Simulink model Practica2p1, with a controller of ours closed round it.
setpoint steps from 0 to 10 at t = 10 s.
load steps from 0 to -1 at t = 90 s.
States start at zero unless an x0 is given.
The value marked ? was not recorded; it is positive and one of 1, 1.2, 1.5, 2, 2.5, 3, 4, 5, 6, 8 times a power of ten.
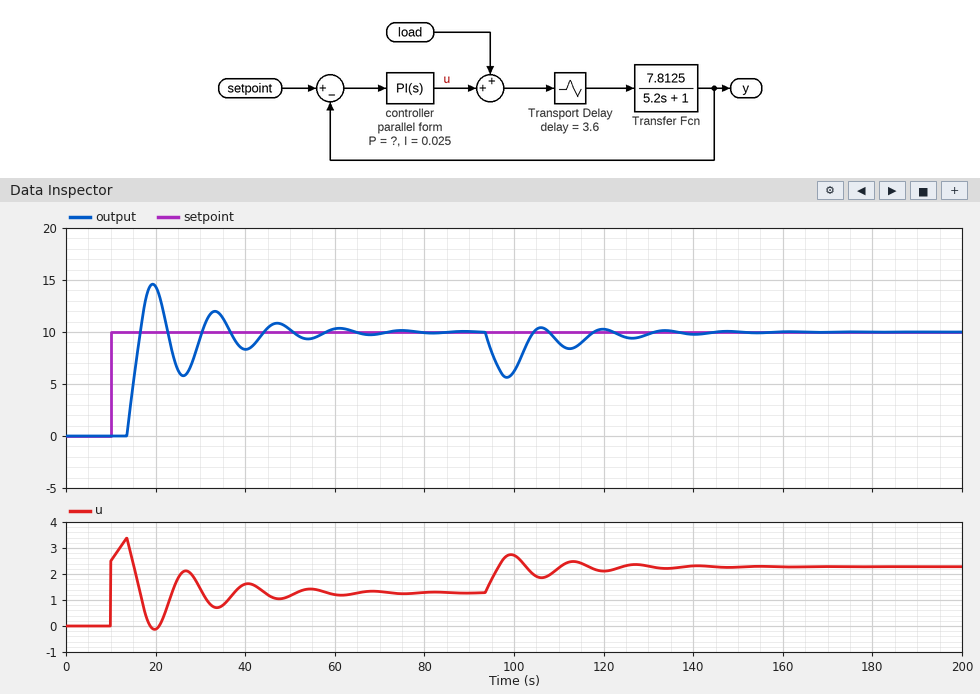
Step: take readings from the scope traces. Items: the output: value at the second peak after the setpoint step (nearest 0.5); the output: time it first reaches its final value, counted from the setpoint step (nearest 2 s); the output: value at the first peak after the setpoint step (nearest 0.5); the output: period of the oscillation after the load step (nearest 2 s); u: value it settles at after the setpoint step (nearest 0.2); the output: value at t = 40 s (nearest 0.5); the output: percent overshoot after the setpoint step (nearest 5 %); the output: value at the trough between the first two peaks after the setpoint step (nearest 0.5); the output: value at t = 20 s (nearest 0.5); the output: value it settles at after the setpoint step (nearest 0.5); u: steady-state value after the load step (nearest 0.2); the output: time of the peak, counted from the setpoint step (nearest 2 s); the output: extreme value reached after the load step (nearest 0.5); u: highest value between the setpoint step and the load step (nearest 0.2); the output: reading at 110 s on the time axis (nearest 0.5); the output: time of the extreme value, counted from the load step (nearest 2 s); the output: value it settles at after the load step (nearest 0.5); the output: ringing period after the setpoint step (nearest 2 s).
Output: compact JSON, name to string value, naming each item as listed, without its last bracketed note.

{"the output: value at the second peak after the setpoint step": "12.0", "the output: time it first reaches its final value, counted from the setpoint step": "6 s", "the output: value at the first peak after the setpoint step": "14.5", "the output: period of the oscillation after the load step": "14 s", "u: value it settles at after the setpoint step": "1.2", "the output: value at t = 40 s": "8.5", "the output: percent overshoot after the setpoint step": "45 %", "the output: value at the trough between the first two peaks after the setpoint step": "6.0", "the output: value at t = 20 s": "14.5", "the output: value it settles at after the setpoint step": "10.0", "u: steady-state value after the load step": "2.2", "the output: time of the peak, counted from the setpoint step": "10 s", "the output: extreme value reached after the load step": "5.5", "u: highest value between the setpoint step and the load step": "3.4", "the output: reading at 110 s on the time axis": "9.0", "the output: time of the extreme value, counted from the load step": "8 s", "the output: value it settles at after the load step": "10.0", "the output: ringing period after the setpoint step": "14 s"}
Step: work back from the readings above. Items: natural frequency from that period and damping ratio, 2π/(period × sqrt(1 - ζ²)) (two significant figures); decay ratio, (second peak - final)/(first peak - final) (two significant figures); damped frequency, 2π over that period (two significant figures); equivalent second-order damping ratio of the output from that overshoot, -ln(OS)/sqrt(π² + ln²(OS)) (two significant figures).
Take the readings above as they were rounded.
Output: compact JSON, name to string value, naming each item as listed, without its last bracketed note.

{"natural frequency from that period and damping ratio, 2π/(period × sqrt(1 - ζ²))": "0.46 rad/s", "decay ratio, (second peak - final)/(first peak - final)": "0.44", "damped frequency, 2π over that period": "0.45 rad/s", "equivalent second-order damping ratio of the output from that overshoot, -ln(OS)/sqrt(π² + ln²(OS))": "0.25"}
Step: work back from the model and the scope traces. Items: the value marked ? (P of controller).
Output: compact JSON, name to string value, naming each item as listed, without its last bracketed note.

{"the value marked ?": "0.25"}
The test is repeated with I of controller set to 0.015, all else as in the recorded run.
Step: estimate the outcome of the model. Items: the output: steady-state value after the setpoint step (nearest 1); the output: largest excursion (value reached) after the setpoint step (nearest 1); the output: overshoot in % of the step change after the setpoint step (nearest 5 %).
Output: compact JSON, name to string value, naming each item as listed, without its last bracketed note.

{"the output: steady-state value after the setpoint step": "10", "the output: largest excursion (value reached) after the setpoint step": "13", "the output: overshoot in % of the step change after the setpoint step": "30 %"}
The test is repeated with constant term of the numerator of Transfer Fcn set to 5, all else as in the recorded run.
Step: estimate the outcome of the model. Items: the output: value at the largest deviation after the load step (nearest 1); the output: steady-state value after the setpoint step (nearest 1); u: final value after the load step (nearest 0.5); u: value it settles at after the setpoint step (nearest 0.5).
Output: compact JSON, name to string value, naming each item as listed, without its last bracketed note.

{"the output: value at the largest deviation after the load step": "7", "the output: steady-state value after the setpoint step": "10", "u: final value after the load step": "3.0", "u: value it settles at after the setpoint step": "2.0"}
